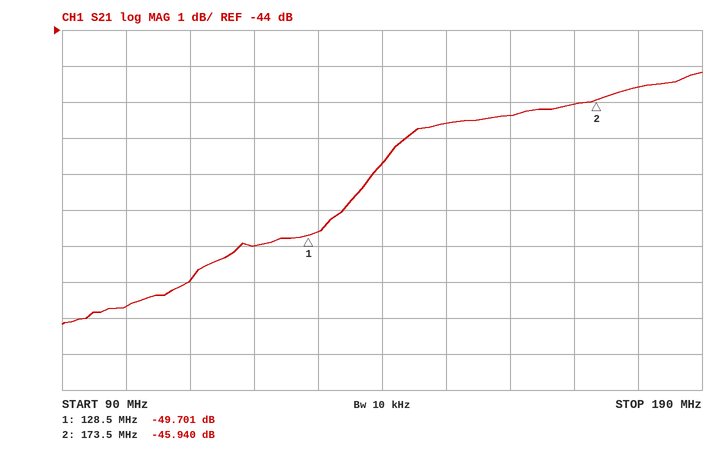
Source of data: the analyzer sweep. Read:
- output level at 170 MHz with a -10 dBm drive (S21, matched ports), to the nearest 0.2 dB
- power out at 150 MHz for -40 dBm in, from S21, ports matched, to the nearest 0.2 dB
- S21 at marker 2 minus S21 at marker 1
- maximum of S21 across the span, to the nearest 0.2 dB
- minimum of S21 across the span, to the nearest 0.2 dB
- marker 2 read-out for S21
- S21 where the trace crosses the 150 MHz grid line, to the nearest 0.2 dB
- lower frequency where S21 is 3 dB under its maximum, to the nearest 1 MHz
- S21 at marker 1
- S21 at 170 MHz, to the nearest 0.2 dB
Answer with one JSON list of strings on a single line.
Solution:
["-56.0 dBm", "-86.6 dBm", "3.761 dB", "-45.2 dB", "-52.2 dB", "-45.940 dB", "-46.6 dB", "138 MHz", "-49.701 dB", "-46.0 dB"]
